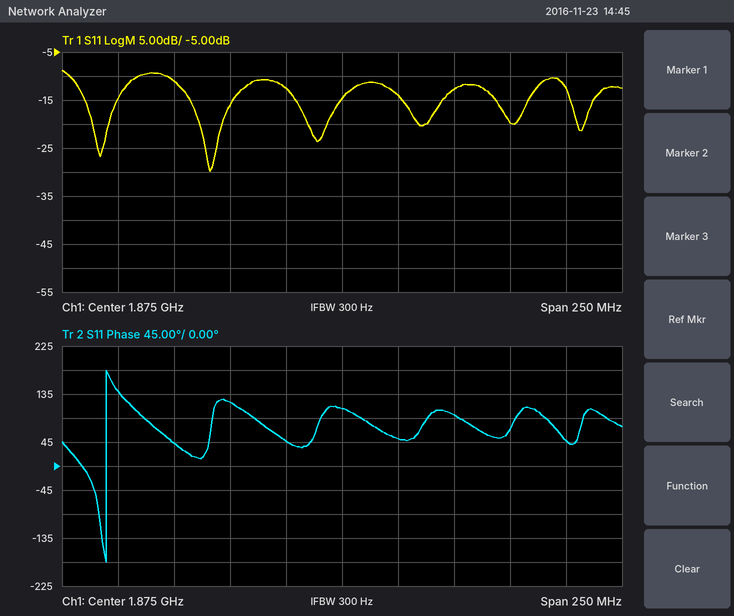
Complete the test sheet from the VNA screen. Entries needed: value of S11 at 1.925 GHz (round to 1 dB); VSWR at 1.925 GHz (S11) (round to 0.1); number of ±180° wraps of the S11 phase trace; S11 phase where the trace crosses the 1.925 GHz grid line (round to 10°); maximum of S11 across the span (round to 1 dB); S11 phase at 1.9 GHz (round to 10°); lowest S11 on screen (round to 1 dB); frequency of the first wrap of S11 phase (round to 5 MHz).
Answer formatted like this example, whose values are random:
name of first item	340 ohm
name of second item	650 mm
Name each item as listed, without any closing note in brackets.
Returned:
value of S11 at 1.925 GHz	-13 dB
VSWR at 1.925 GHz (S11)	1.6
number of ±180° wraps of the S11 phase trace	1
S11 phase where the trace crosses the 1.925 GHz grid line	100°
maximum of S11 across the span	-9 dB
S11 phase at 1.9 GHz	50°
lowest S11 on screen	-30 dB
frequency of the first wrap of S11 phase	1.770 GHz
